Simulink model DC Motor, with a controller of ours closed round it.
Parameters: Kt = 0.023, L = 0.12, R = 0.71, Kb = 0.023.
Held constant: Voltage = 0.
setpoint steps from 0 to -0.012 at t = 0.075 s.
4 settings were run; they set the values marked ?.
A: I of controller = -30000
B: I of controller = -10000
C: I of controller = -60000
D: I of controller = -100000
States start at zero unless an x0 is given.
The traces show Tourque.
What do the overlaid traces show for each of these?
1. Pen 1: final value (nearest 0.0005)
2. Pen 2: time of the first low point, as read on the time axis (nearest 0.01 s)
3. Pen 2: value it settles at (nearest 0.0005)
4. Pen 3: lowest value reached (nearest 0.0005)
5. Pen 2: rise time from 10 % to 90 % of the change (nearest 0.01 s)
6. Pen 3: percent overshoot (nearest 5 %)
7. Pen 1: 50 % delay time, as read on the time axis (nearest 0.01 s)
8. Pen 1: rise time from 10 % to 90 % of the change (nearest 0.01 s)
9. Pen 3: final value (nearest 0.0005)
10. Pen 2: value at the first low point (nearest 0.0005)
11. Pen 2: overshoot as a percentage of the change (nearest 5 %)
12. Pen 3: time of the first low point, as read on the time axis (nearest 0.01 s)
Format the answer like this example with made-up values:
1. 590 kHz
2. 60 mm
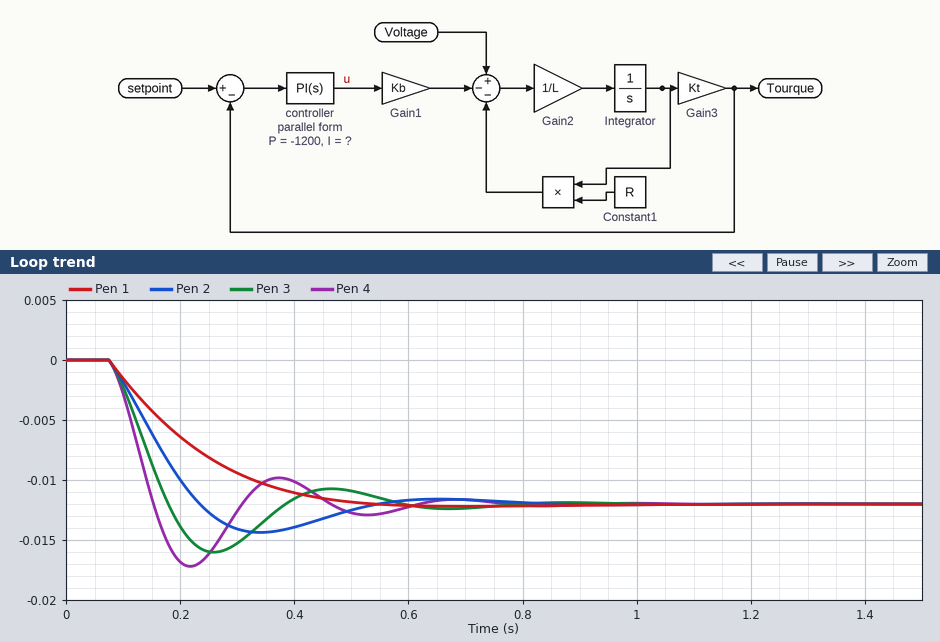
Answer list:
1. -0.0120
2. 0.34 s
3. -0.0120
4. -0.0160
5. 0.12 s
6. 35 %
7. 0.19 s
8. 0.28 s
9. -0.0120
10. -0.0145
11. 20 %
12. 0.26 s
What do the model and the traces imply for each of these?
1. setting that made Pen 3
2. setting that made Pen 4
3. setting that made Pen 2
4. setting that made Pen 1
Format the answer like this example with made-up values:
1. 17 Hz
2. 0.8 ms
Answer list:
1. C
2. D
3. A
4. B
